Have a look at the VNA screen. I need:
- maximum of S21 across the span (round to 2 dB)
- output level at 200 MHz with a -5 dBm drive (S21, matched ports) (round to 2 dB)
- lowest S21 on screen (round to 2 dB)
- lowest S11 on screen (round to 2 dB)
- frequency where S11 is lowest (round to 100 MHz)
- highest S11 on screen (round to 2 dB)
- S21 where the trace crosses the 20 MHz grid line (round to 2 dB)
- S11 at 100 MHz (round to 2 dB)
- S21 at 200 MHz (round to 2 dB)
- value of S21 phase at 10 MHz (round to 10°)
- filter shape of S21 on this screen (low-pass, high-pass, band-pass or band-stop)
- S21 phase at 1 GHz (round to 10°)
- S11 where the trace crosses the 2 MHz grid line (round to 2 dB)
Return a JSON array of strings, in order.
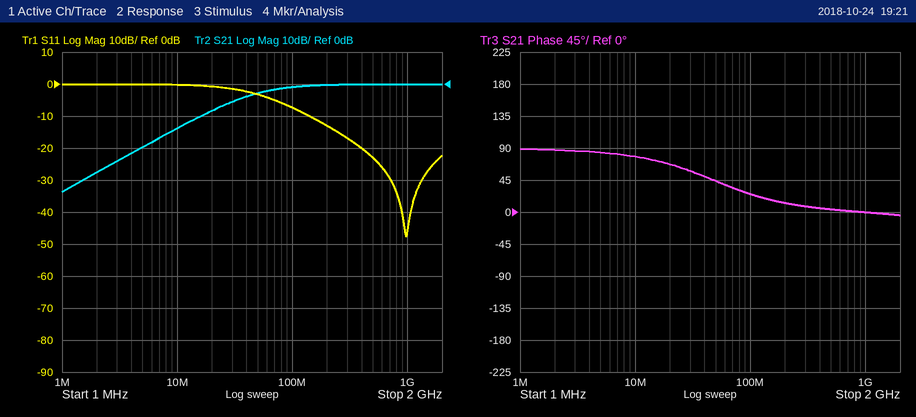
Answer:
["0 dB", "-6 dBm", "-34 dB", "-48 dB", "1.0 GHz", "0 dB", "-8 dB", "-8 dB", "0 dB", "80°", "high-pass", "0°", "0 dB"]
